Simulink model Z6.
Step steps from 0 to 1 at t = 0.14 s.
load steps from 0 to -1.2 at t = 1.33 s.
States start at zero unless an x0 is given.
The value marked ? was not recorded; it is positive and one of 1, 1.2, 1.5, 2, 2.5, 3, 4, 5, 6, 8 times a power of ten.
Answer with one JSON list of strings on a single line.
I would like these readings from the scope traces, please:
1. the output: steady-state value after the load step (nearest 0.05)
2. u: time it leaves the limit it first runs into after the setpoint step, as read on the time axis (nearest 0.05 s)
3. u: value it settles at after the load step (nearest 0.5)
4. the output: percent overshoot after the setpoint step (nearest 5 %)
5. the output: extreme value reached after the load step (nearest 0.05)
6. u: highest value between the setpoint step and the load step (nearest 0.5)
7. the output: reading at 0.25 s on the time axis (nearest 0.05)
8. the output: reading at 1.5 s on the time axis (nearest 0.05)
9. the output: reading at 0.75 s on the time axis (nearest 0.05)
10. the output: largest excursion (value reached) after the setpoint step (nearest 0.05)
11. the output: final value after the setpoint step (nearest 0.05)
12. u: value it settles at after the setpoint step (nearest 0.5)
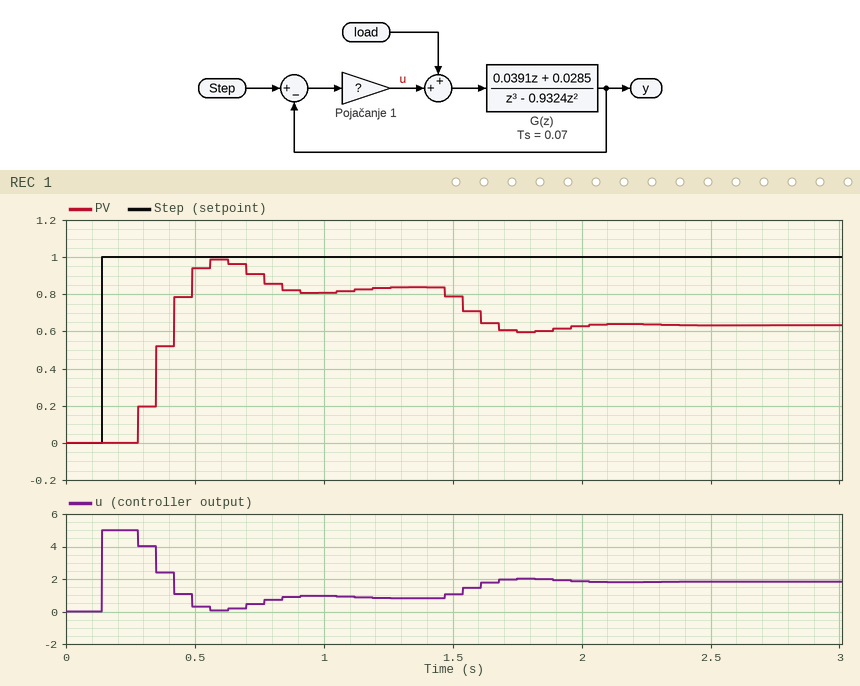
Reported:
["0.65", "0.30 s", "2.0", "20 %", "0.60", "5.0", "0.00", "0.80", "0.90", "1.00", "0.85", "1.0"]
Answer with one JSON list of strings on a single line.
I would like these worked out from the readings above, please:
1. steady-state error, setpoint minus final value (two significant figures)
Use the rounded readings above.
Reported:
["0.15"]
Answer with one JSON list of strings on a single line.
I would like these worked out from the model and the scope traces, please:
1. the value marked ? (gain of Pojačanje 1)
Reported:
["5"]
